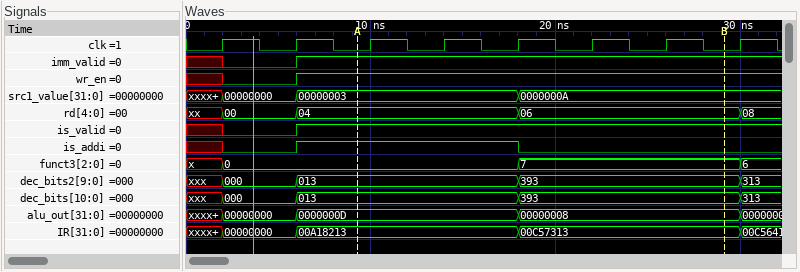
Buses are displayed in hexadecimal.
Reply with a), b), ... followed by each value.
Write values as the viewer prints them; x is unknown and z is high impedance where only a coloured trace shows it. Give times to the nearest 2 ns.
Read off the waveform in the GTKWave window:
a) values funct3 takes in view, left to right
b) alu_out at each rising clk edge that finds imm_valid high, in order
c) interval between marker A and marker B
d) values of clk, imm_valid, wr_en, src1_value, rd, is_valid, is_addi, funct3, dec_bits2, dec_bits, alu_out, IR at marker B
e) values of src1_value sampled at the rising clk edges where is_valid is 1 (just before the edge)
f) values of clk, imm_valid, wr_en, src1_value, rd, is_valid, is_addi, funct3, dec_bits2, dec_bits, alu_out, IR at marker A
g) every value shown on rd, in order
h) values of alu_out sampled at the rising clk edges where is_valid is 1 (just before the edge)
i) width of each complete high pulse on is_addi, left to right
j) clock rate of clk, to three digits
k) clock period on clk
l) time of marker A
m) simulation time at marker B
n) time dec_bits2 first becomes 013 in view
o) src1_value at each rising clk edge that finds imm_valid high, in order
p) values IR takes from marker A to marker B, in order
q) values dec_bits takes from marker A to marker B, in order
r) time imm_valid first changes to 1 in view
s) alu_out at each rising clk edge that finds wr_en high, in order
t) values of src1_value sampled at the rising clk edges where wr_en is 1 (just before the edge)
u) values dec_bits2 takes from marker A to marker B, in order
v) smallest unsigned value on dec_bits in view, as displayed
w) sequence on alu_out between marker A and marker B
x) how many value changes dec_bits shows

a) x, 0, 7, 6
b) 0000000D, 0000000D, 0000000D, 00000008, 00000008, 00000008
c) 20 ns
d) clk=0, imm_valid=1, wr_en=1, src1_value=0000000A, rd=06, is_valid=1, is_addi=0, funct3=7, dec_bits2=393, dec_bits=393, alu_out=00000008, IR=00C57313
e) 00000003, 00000003, 00000003, 0000000A, 0000000A, 0000000A
f) clk=0, imm_valid=1, wr_en=1, src1_value=00000003, rd=04, is_valid=1, is_addi=1, funct3=0, dec_bits2=013, dec_bits=013, alu_out=0000000D, IR=00A18213
g) xx, 00, 04, 06, 08
h) 0000000D, 0000000D, 0000000D, 00000008, 00000008, 00000008
i) 12 ns
j) 250 MHz
k) 4 ns
l) 10 ns
m) 30 ns
n) 6 ns
o) 00000003, 00000003, 00000003, 0000000A, 0000000A, 0000000A
p) 00A18213, 00C57313
q) 013, 393
r) 6 ns
s) 0000000D, 0000000D, 0000000D, 00000008, 00000008, 00000008
t) 00000003, 00000003, 00000003, 0000000A, 0000000A, 0000000A
u) 013, 393
v) 000
w) 0000000D, 00000008
x) 4
